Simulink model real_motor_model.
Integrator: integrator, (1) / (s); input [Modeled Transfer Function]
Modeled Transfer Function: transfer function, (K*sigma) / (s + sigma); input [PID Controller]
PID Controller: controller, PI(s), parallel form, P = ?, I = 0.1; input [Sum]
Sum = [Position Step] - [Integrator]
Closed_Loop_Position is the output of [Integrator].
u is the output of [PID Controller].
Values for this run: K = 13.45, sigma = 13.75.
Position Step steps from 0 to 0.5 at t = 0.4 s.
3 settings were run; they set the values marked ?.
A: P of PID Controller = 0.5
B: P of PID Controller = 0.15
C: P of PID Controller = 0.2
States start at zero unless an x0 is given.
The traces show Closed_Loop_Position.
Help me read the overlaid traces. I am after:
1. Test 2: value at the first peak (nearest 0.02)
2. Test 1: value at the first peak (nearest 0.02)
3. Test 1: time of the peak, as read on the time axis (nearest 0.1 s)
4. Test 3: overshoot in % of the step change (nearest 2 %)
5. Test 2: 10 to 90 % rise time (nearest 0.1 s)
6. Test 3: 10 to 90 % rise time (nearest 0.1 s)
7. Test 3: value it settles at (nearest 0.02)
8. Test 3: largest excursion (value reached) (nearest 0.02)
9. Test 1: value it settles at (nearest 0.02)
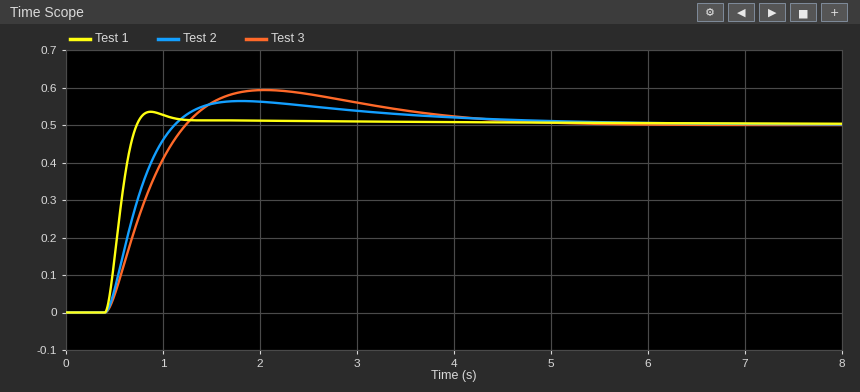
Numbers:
0.56
0.54
0.9 s
18 %
0.5 s
0.6 s
0.50
0.60
0.50
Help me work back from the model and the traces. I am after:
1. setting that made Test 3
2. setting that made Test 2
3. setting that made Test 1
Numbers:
B
C
A
